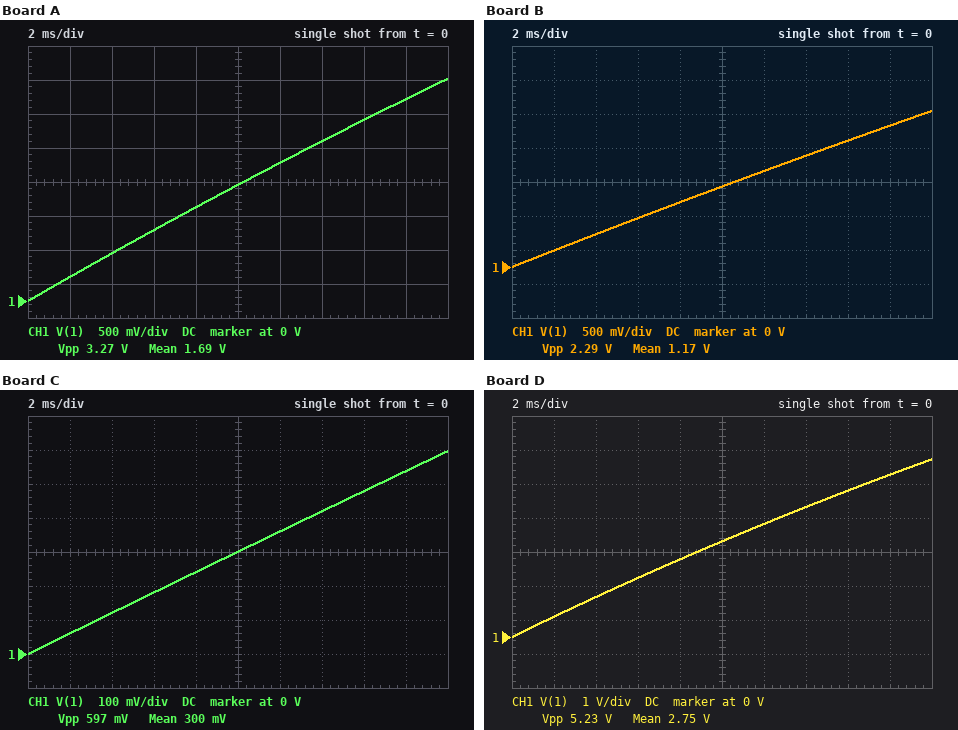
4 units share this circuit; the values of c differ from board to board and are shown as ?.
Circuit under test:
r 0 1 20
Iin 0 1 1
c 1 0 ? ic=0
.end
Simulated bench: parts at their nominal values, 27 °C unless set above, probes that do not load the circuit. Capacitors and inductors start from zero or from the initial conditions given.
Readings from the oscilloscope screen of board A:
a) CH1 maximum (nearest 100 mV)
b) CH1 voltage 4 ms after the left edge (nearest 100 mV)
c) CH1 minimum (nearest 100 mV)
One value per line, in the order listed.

3.3 V
700 mV
0 V
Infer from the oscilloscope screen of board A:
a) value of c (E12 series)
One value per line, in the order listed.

5.6 mF
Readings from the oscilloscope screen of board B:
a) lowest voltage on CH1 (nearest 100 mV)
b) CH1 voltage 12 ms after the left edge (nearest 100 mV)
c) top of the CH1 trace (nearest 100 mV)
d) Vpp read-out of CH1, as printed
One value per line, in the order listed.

0 V
1.4 V
2.3 V
2.29 V
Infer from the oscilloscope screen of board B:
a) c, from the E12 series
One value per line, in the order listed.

8.2 mF
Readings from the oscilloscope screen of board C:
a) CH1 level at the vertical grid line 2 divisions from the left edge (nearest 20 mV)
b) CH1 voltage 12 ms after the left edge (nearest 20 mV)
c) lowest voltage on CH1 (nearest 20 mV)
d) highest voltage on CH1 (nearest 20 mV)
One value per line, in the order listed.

120 mV
360 mV
0 V
600 mV
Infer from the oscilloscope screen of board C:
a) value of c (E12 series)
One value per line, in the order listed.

33 mF
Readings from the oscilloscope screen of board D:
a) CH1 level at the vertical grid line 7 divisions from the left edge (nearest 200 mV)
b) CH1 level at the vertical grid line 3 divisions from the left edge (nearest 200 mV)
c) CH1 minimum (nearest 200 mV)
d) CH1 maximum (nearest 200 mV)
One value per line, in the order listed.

3.8 V
1.8 V
0 V
5.2 V
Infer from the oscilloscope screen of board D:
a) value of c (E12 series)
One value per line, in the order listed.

3.3 mF
